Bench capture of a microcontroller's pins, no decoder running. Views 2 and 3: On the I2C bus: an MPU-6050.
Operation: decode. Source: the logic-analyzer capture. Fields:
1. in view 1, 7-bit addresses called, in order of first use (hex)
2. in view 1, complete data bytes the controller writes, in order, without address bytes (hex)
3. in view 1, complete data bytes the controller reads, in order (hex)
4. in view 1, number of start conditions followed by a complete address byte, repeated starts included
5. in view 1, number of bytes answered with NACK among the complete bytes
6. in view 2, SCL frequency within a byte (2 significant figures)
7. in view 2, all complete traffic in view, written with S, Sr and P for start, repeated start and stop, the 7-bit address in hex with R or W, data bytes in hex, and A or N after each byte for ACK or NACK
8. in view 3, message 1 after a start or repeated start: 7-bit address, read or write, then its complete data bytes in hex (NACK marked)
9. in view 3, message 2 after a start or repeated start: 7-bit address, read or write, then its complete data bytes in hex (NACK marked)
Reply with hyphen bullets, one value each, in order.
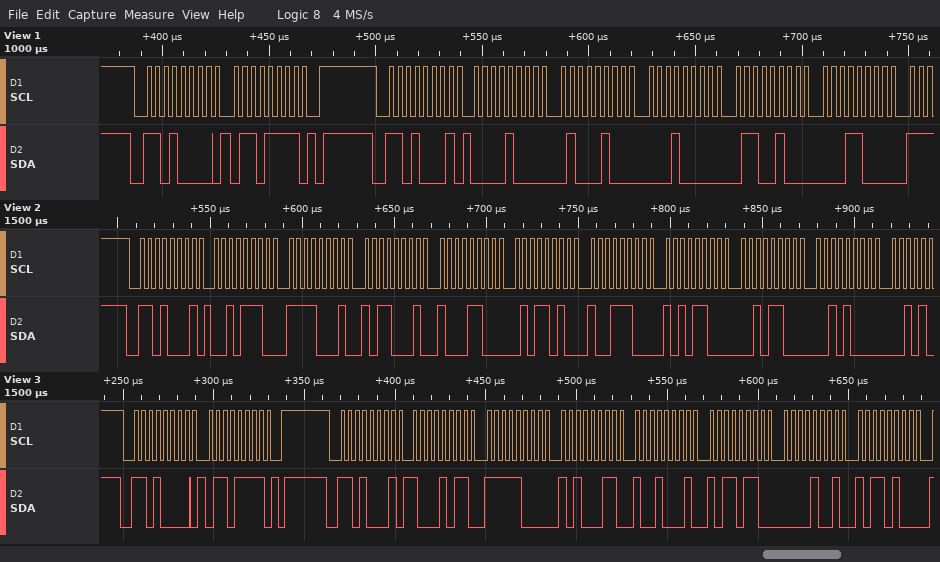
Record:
- 0x68
- 6F
- 08 44 10 64 18
- 2
- 0
- 250 kHz
- S 68R A 2E A F1 A B1 A 8C A 5A A 9C A AC A 2C A 28 A
- 0x68 write: 6F
- 0x68 read: 8B F8 A3 91 B6 09 B4
